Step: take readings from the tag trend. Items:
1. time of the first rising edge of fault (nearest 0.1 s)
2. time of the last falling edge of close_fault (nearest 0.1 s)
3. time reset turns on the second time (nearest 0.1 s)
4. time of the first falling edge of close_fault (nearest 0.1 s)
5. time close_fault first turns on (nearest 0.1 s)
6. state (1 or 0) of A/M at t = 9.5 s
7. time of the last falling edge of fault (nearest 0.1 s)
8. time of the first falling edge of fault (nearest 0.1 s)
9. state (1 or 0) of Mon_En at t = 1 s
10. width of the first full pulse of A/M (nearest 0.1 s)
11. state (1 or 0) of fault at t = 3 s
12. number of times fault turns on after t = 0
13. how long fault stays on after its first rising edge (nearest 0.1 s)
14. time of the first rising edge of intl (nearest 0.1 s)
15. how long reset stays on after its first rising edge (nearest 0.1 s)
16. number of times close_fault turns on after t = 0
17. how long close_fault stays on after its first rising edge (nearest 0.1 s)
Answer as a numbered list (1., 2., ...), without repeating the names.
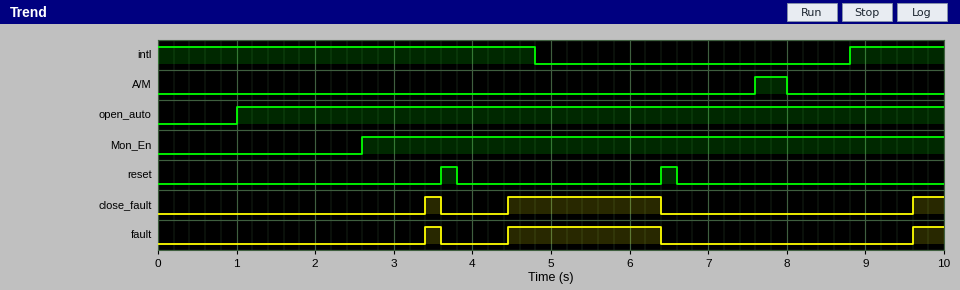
1. 3.4 s
2. 6.4 s
3. 6.4 s
4. 3.6 s
5. 3.4 s
6. 0
7. 6.4 s
8. 3.6 s
9. 0
10. 0.4 s
11. 0
12. 3
13. 0.2 s
14. 8.8 s
15. 0.2 s
16. 3
17. 0.2 s
